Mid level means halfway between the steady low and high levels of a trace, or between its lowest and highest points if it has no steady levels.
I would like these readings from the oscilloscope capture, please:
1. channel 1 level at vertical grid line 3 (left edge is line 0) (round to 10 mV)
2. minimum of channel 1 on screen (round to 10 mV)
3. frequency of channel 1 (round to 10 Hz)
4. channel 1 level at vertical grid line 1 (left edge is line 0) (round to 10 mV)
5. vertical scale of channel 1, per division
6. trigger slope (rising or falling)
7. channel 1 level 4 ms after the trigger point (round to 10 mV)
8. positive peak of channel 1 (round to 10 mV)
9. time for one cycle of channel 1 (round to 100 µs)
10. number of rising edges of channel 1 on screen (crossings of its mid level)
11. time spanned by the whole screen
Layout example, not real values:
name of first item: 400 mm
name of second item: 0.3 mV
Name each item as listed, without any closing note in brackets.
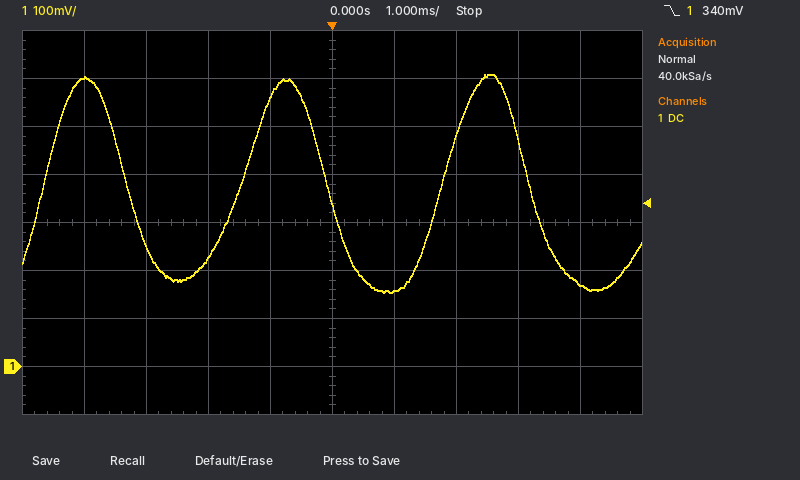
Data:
channel 1 level at vertical grid line 3 (left edge is line 0): 230 mV
minimum of channel 1 on screen: 150 mV
frequency of channel 1: 310 Hz
channel 1 level at vertical grid line 1 (left edge is line 0): 600 mV
vertical scale of channel 1, per division: 100 mV
trigger slope: falling
channel 1 level 4 ms after the trigger point: 170 mV
positive peak of channel 1: 610 mV
time for one cycle of channel 1: 3.2 ms
number of rising edges of channel 1 on screen: 3
time spanned by the whole screen: 10 ms
